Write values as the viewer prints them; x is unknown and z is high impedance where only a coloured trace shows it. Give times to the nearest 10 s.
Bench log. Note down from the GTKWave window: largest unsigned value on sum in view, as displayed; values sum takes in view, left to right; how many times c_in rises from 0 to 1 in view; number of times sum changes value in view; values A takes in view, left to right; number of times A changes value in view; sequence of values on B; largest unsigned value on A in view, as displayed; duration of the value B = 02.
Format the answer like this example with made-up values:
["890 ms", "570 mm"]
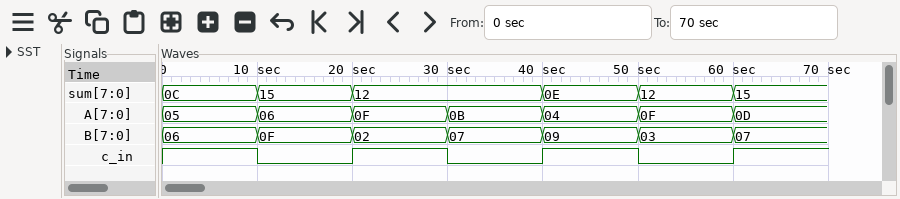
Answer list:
["15", "0C, 15, 12, 0E, 12, 15", "3", "5", "05, 06, 0F, 0B, 04, 0F, 0D", "6", "06, 0F, 02, 07, 09, 03, 07", "0F", "10 s"]
